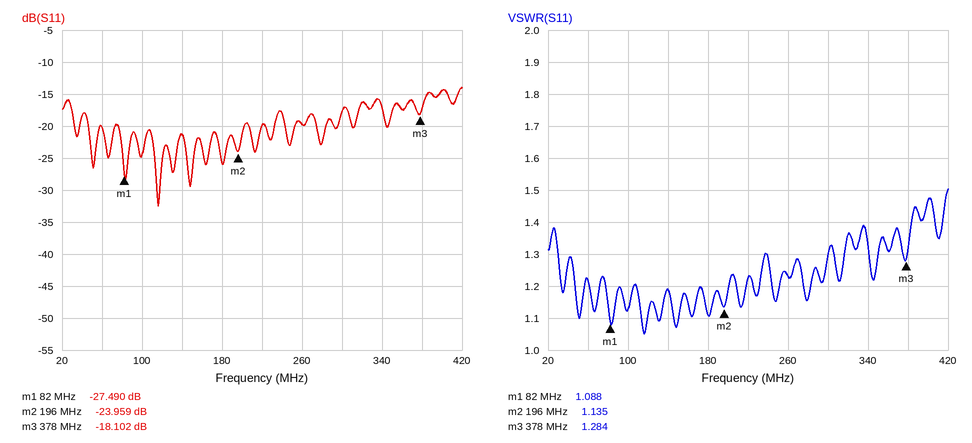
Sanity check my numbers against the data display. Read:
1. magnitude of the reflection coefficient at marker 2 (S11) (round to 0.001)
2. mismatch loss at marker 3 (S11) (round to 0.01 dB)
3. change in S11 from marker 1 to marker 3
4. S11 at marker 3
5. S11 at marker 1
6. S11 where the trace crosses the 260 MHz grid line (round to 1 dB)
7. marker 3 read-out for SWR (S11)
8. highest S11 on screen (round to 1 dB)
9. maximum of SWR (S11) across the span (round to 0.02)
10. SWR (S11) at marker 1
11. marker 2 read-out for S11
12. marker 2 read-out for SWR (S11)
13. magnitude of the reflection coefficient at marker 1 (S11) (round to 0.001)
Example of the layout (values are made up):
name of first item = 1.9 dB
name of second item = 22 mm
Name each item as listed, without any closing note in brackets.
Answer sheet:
magnitude of the reflection coefficient at marker 2 (S11) = 0.063
mismatch loss at marker 3 (S11) = 0.07 dB
change in S11 from marker 1 to marker 3 = 9.388 dB
S11 at marker 3 = -18.102 dB
S11 at marker 1 = -27.490 dB
S11 where the trace crosses the 260 MHz grid line = -20 dB
marker 3 read-out for SWR = 1.284
highest S11 on screen = -14 dB
maximum of SWR (S11) across the span = 1.50
SWR (S11) at marker 1 = 1.088
marker 2 read-out for S11 = -23.959 dB
marker 2 read-out for SWR = 1.135
magnitude of the reflection coefficient at marker 1 (S11) = 0.042
